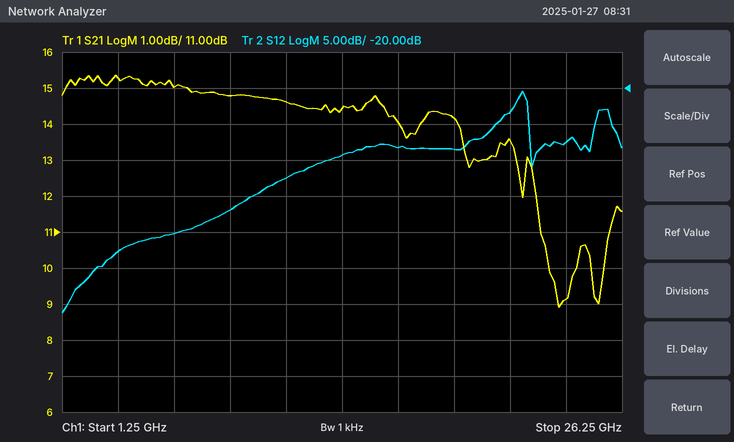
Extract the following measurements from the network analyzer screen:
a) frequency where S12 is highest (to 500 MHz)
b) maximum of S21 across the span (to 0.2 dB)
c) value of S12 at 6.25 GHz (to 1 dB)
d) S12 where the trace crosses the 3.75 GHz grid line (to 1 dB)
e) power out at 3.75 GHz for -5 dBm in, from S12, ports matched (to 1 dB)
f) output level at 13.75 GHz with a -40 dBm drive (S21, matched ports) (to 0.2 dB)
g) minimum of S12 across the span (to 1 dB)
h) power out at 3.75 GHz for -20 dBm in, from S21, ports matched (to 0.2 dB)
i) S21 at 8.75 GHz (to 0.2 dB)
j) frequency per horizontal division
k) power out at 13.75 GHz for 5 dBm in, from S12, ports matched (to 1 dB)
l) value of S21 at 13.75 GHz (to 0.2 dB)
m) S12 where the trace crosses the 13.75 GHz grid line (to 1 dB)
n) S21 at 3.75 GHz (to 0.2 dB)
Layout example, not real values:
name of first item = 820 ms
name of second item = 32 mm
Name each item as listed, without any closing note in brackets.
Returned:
frequency where S12 is highest = 22.0 GHz
maximum of S21 across the span = 15.4 dB
value of S12 at 6.25 GHz = -40 dB
S12 where the trace crosses the 3.75 GHz grid line = -43 dB
power out at 3.75 GHz for -5 dBm in, from S12, ports matched = -48 dBm
output level at 13.75 GHz with a -40 dBm drive (S21, matched ports) = -25.6 dBm
minimum of S12 across the span = -51 dB
power out at 3.75 GHz for -20 dBm in, from S21, ports matched = -4.8 dBm
S21 at 8.75 GHz = 14.8 dB
frequency per horizontal division = 2.5 GHz
power out at 13.75 GHz for 5 dBm in, from S12, ports matched = -24 dBm
value of S21 at 13.75 GHz = 14.4 dB
S12 where the trace crosses the 13.75 GHz grid line = -29 dB
S21 at 3.75 GHz = 15.2 dB
